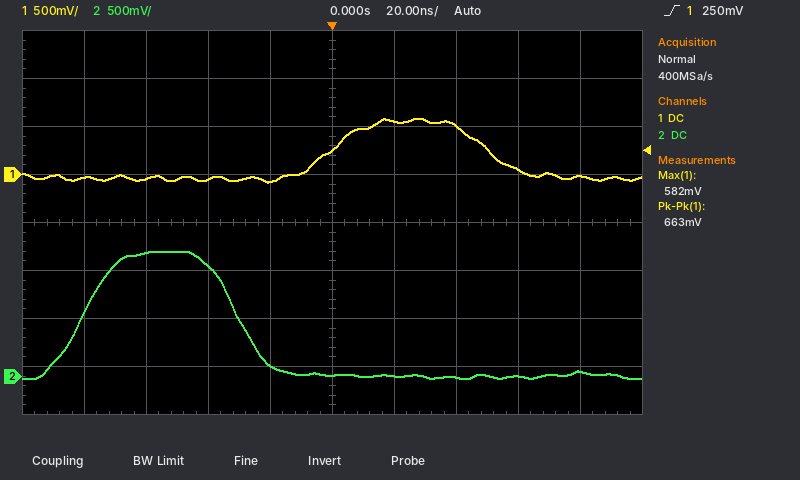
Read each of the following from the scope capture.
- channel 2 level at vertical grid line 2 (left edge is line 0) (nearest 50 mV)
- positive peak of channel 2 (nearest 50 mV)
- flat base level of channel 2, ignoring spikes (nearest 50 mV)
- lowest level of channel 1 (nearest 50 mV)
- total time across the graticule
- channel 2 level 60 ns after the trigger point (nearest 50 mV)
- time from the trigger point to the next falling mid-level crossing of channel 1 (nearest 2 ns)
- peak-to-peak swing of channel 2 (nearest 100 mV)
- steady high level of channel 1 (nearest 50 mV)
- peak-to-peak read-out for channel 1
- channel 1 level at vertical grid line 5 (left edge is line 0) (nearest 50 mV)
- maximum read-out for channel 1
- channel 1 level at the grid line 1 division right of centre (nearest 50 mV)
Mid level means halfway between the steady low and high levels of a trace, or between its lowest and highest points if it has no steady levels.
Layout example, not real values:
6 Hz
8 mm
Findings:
1.30 V
1.30 V
0 mV
-100 mV
200 ns
0 mV
50 ns
1.30 V
550 mV
663 mV
250 mV
582 mV
550 mV
